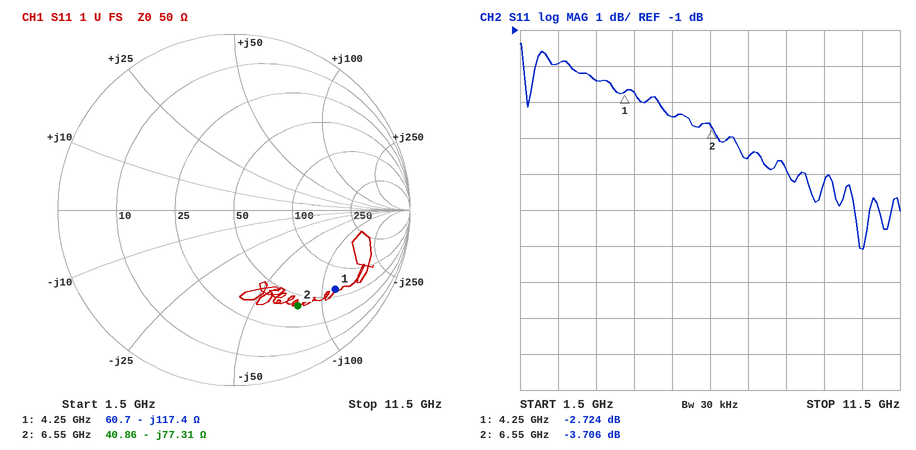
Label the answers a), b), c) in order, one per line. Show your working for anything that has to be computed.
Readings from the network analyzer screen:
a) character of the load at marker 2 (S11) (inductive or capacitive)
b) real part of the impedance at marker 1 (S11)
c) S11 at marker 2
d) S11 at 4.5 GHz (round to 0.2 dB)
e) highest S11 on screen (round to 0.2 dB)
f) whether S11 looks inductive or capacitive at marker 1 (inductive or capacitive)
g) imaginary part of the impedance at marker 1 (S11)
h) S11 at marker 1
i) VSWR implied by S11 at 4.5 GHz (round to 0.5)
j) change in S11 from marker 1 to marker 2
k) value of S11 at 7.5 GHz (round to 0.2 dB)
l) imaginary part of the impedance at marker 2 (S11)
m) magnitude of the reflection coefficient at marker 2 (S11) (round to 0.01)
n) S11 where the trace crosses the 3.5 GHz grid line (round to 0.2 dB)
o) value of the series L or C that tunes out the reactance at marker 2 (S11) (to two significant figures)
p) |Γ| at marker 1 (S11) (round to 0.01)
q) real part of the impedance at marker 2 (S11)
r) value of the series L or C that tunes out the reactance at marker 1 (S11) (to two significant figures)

a) capacitive
b) 60.7 Ω
c) -3.706 dB
d) -2.8 dB
e) -1.4 dB
f) capacitive
g) -117.4 Ω
h) -2.724 dB
i) |Γ| = 10^(-2.8/20) = 0.7244; VSWR = (1 + 0.7244)/(1 − 0.7244) ≈ 6.26, so 6.5 to the nearest 0.5
j) -3.706 − (-2.724) = -0.982 dB
k) -4.6 dB
l) -77.31 Ω
m) 0.65
n) -2.4 dB
o) L = 77.31 Ω/(2π × 6.55 GHz) ≈ 1.9 nH
p) 0.73
q) 40.86 Ω
r) L = 117.4 Ω/(2π × 4.25 GHz) ≈ 4.4 nH
